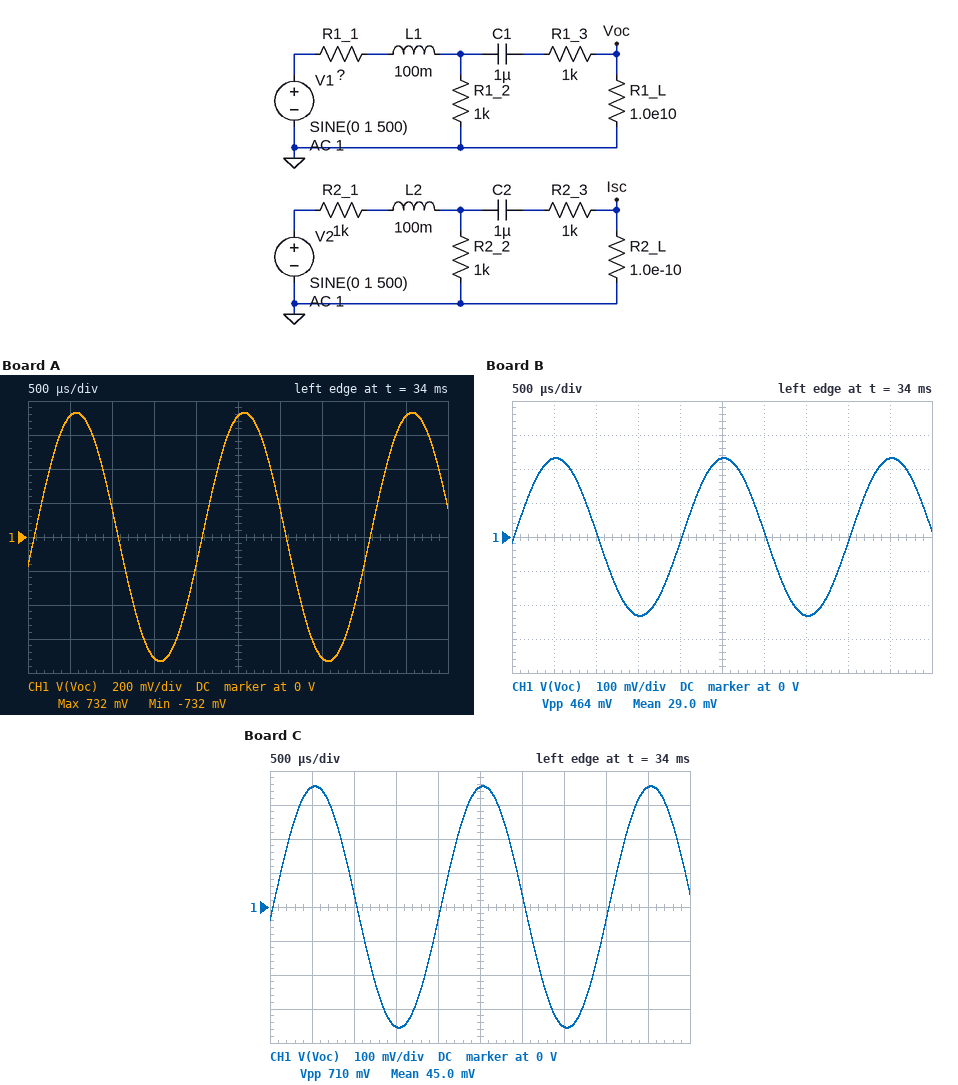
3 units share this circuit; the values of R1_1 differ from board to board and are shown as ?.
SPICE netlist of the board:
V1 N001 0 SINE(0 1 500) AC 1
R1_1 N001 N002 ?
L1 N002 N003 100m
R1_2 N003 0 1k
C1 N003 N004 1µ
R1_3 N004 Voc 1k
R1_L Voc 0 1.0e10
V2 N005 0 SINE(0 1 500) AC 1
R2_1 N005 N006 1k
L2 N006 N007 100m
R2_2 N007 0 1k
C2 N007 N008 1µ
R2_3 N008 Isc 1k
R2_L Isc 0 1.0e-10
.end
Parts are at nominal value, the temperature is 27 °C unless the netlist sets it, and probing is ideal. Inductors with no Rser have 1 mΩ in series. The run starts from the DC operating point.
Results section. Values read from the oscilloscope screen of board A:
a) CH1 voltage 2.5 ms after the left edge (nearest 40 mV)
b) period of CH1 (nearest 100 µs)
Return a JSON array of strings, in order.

["720 mV", "2.0 ms"]
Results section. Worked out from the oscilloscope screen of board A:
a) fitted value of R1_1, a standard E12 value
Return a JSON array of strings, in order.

["330 Ω"]
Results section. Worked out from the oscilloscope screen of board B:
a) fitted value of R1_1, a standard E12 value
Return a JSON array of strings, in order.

["3.3 kΩ"]
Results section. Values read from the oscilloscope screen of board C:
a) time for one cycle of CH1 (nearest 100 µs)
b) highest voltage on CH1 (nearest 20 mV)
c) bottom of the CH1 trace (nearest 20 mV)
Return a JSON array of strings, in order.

["2.0 ms", "360 mV", "-360 mV"]
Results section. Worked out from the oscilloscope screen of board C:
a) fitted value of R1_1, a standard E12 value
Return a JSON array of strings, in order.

["1.8 kΩ"]
